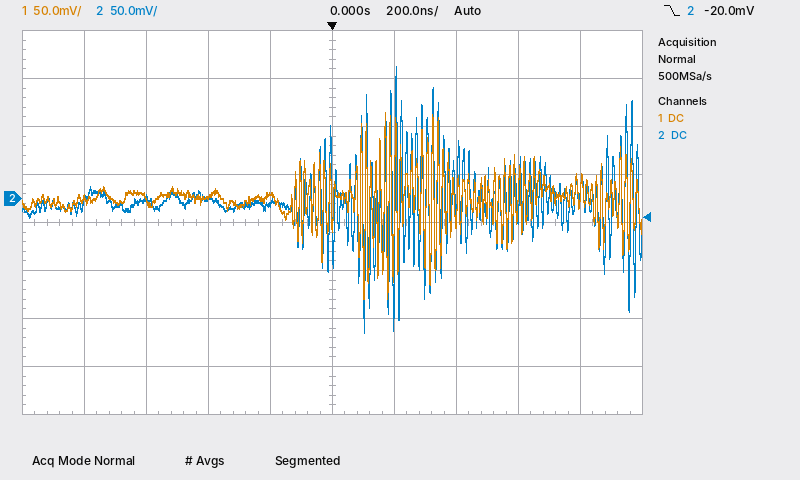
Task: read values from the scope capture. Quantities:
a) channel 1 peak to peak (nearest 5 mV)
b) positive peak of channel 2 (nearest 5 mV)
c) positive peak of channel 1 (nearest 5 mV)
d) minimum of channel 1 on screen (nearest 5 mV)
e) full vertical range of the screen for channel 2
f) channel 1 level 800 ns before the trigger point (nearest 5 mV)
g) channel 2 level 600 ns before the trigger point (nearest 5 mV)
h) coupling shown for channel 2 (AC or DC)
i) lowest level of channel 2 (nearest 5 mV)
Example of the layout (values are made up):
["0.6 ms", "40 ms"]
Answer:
["195 mV", "140 mV", "90 mV", "-105 mV", "400 mV", "0 mV", "0 mV", "DC", "-140 mV"]
